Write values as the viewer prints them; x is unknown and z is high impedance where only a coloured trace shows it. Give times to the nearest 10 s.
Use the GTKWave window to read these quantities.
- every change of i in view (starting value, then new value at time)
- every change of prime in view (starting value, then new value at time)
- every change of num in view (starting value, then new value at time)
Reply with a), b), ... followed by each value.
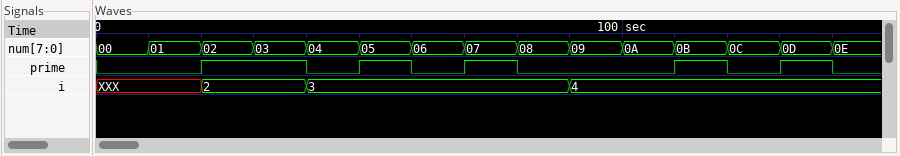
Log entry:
a) XXX, 2 at 20 s, 3 at 40 s, 4 at 90 s
b) 0, 1 at 20 s, 0 at 40 s, 1 at 50 s, 0 at 60 s, 1 at 70 s, 0 at 80 s, 1 at 110 s, 0 at 120 s, 1 at 130 s, 0 at 140 s
c) 00, 01 at 10 s, 02 at 20 s, 03 at 30 s, 04 at 40 s, 05 at 50 s, 06 at 60 s, 07 at 70 s, 08 at 80 s, 09 at 90 s, 0A at 100 s, 0B at 110 s, 0C at 120 s, 0D at 130 s, 0E at 140 s
